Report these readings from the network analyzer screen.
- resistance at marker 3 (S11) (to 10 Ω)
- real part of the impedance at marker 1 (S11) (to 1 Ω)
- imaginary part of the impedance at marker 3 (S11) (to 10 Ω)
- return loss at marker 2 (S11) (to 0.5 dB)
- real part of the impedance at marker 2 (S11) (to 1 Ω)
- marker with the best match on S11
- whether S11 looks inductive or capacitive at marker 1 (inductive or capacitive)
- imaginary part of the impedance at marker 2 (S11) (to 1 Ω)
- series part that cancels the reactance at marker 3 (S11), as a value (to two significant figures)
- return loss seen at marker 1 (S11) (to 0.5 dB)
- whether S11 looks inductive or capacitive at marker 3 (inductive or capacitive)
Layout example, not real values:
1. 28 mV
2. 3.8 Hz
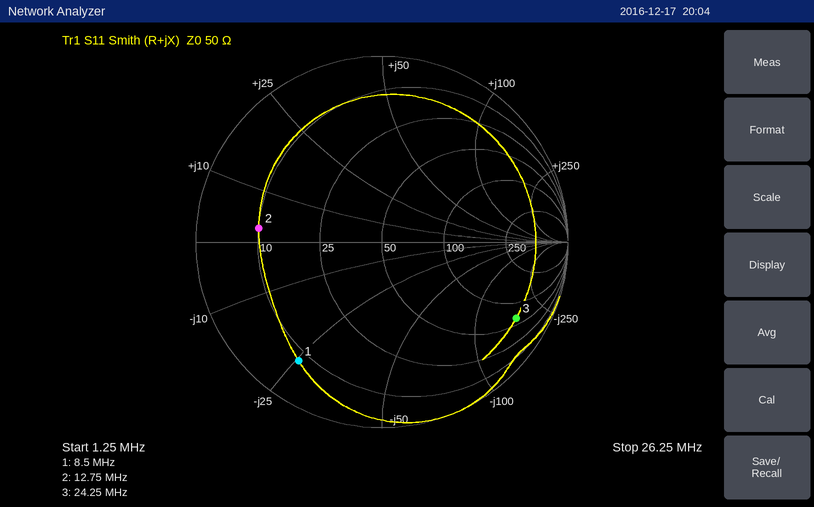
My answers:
1. 60 Ω
2. 8 Ω
3. -170 Ω
4. 3.5 dB
5. 10 Ω
6. marker 2
7. capacitive
8. +3 Ω
9. 1.1 µH
10. 2.0 dB
11. capacitive
